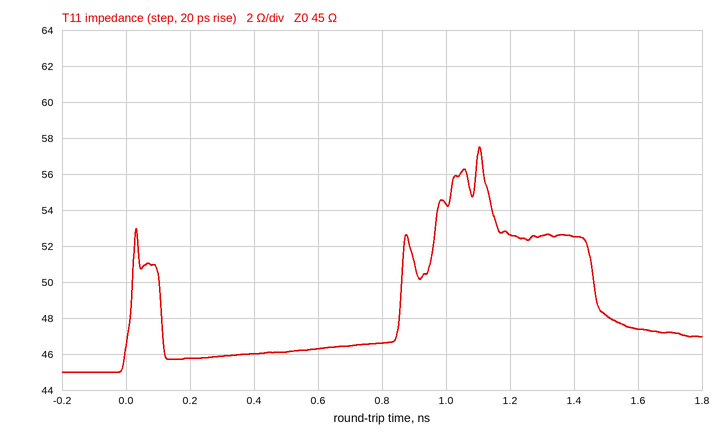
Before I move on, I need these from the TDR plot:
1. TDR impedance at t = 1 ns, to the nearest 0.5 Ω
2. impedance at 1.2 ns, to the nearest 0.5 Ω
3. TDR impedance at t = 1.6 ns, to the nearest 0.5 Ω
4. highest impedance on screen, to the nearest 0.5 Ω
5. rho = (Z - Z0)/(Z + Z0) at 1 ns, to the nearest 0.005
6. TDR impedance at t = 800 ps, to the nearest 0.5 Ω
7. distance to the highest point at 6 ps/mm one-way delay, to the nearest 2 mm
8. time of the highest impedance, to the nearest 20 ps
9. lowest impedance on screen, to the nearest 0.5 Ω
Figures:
54.5 Ω
52.5 Ω
47.5 Ω
57.5 Ω
+0.095
46.5 Ω
92 mm
1.10 ns
45.0 Ω
